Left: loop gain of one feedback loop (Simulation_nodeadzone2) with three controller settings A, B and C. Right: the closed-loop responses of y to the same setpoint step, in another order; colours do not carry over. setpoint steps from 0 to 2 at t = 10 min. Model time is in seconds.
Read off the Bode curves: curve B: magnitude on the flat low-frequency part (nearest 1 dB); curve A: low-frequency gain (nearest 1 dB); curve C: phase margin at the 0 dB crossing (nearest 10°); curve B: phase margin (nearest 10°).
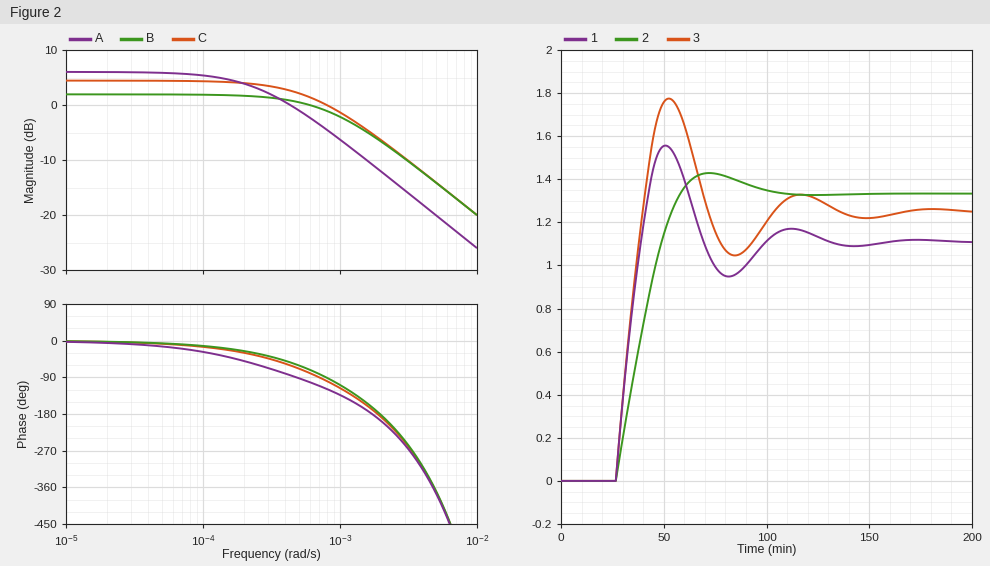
2 dB
6 dB
80°
110°
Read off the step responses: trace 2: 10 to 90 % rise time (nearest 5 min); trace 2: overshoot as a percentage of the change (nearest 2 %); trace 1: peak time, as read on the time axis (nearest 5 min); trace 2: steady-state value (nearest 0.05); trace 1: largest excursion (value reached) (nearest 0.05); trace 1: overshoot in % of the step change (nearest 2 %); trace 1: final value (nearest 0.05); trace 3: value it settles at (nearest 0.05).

25 min
8 %
50 min
1.35
1.55
40 %
1.10
1.25
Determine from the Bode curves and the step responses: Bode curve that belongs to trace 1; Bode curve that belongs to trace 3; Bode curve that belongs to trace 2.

B
C
A
